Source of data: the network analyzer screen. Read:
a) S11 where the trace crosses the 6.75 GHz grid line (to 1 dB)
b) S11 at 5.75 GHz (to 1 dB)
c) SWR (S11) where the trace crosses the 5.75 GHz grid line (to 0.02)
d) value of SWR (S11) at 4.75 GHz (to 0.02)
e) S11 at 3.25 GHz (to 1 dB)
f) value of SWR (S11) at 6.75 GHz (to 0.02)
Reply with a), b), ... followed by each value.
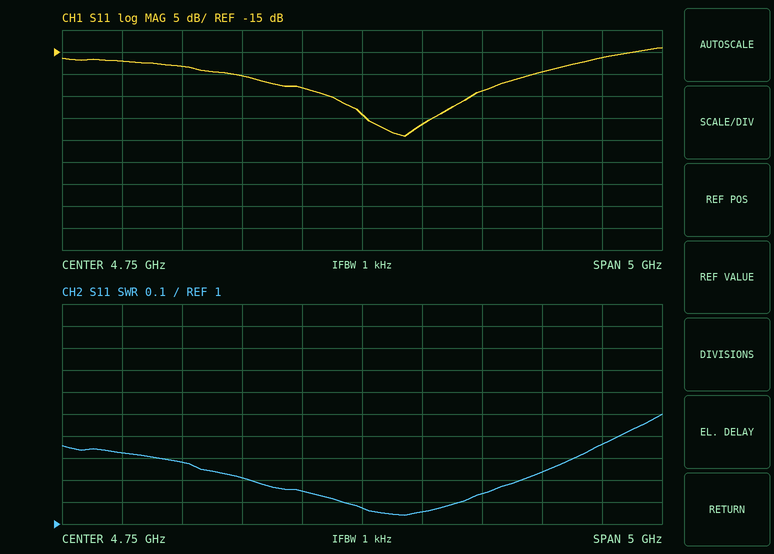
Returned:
a) -16 dB
b) -24 dB
c) 1.14
d) 1.08
e) -18 dB
f) 1.36
